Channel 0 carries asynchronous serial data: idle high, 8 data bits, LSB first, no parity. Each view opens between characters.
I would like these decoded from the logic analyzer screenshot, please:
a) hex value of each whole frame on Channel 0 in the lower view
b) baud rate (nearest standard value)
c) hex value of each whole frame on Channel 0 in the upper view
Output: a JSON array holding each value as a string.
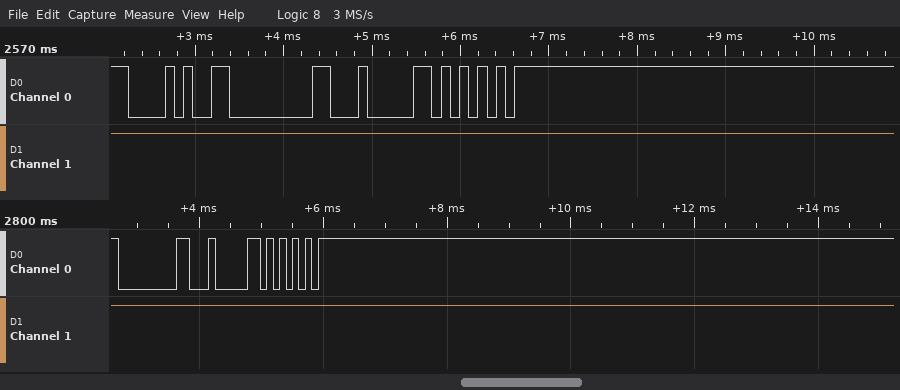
["00, 04, 55", "9600 baud", "28, 00, 04, 55"]
